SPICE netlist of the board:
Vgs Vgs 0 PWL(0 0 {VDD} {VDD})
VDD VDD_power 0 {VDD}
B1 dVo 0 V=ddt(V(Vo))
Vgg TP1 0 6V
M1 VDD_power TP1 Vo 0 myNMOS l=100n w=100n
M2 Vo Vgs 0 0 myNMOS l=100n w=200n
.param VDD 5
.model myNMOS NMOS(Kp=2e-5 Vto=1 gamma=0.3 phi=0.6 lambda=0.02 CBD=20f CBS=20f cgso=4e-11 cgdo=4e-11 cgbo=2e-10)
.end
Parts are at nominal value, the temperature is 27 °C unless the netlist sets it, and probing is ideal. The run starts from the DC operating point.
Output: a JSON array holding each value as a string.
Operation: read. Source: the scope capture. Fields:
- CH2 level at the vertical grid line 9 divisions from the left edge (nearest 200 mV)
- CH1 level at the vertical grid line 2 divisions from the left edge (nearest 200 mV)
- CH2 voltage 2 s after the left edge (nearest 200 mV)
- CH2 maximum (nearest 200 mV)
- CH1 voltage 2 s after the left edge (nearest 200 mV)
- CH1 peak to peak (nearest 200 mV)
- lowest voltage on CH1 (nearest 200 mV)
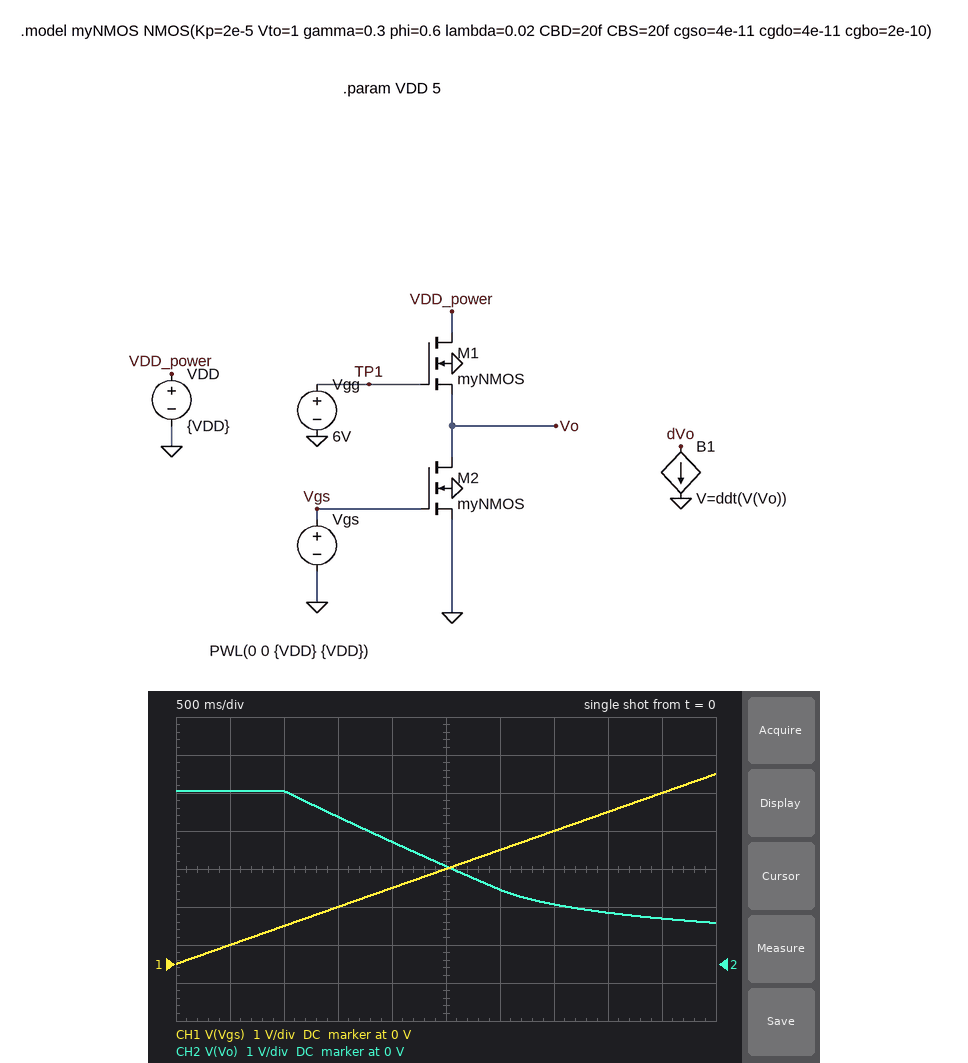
["1.2 V", "1.0 V", "3.2 V", "4.6 V", "2.0 V", "5.0 V", "0 V"]
